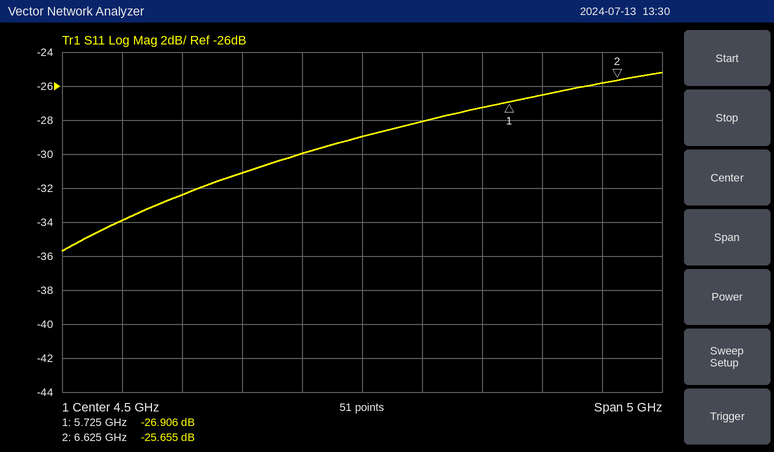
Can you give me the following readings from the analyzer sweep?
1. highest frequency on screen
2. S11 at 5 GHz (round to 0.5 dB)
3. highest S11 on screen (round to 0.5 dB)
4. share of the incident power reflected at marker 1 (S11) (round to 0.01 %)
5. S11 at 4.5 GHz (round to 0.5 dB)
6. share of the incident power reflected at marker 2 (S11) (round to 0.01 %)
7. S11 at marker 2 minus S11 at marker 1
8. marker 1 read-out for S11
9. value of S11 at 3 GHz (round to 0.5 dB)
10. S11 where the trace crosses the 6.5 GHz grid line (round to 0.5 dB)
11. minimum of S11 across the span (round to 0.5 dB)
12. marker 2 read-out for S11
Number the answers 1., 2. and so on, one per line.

1. 7 GHz
2. -28.0 dB
3. -25.0 dB
4. 0.20 %
5. -29.0 dB
6. 0.27 %
7. 1.251 dB
8. -26.906 dB
9. -32.5 dB
10. -26.0 dB
11. -35.5 dB
12. -25.655 dB
